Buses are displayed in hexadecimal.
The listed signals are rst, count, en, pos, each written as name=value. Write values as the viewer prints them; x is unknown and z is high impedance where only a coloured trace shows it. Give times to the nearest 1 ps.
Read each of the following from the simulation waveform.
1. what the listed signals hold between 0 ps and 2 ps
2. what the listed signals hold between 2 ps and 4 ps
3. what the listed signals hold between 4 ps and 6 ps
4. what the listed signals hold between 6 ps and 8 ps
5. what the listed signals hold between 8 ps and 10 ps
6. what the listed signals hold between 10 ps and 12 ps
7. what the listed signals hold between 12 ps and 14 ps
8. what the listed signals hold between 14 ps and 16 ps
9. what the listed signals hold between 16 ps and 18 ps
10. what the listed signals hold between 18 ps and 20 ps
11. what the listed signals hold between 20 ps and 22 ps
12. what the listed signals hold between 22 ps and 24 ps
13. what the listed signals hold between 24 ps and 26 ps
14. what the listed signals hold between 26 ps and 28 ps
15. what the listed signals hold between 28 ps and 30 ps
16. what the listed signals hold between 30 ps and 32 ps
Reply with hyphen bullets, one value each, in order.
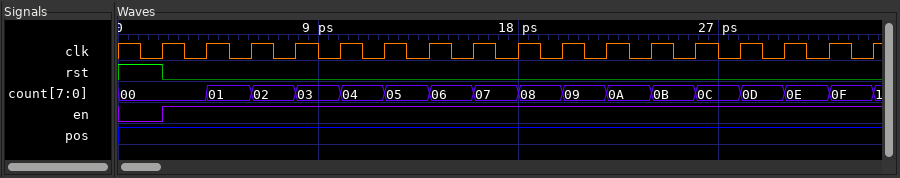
- rst=1, count=00, en=0, pos=1
- rst=0, count=00, en=1, pos=1
- rst=0, count=01, en=1, pos=1
- rst=0, count=02, en=1, pos=1
- rst=0, count=03, en=1, pos=1
- rst=0, count=04, en=1, pos=1
- rst=0, count=05, en=1, pos=1
- rst=0, count=06, en=1, pos=1
- rst=0, count=07, en=1, pos=1
- rst=0, count=08, en=1, pos=1
- rst=0, count=09, en=1, pos=1
- rst=0, count=0A, en=1, pos=1
- rst=0, count=0B, en=1, pos=1
- rst=0, count=0C, en=1, pos=1
- rst=0, count=0D, en=1, pos=1
- rst=0, count=0E, en=1, pos=1
